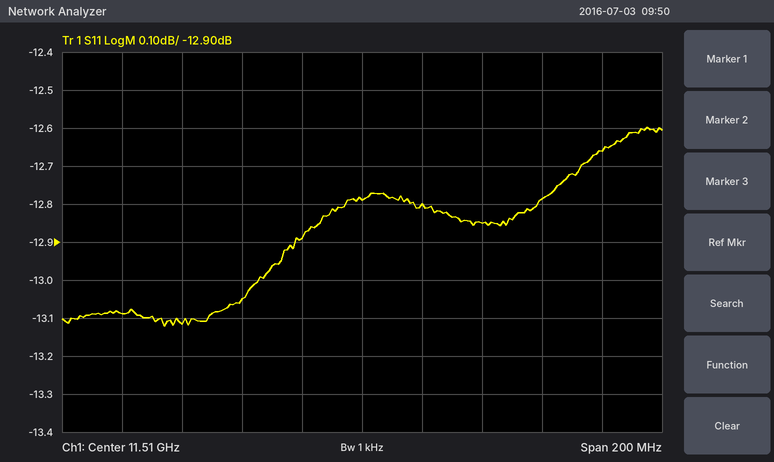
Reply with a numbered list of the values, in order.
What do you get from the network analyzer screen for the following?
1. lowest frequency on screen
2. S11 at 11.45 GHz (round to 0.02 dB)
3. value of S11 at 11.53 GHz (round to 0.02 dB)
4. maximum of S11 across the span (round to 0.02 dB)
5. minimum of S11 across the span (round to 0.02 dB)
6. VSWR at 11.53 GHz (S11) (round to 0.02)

1. 11.41 GHz
2. -13.12 dB
3. -12.80 dB
4. -12.60 dB
5. -13.12 dB
6. 1.60
